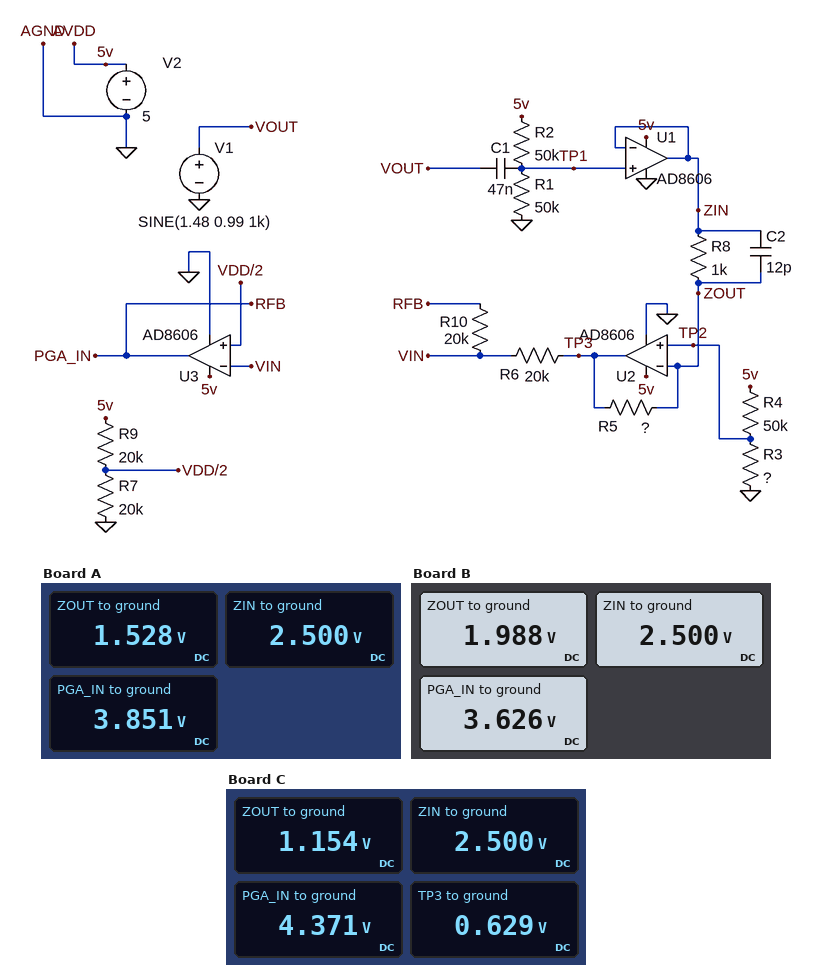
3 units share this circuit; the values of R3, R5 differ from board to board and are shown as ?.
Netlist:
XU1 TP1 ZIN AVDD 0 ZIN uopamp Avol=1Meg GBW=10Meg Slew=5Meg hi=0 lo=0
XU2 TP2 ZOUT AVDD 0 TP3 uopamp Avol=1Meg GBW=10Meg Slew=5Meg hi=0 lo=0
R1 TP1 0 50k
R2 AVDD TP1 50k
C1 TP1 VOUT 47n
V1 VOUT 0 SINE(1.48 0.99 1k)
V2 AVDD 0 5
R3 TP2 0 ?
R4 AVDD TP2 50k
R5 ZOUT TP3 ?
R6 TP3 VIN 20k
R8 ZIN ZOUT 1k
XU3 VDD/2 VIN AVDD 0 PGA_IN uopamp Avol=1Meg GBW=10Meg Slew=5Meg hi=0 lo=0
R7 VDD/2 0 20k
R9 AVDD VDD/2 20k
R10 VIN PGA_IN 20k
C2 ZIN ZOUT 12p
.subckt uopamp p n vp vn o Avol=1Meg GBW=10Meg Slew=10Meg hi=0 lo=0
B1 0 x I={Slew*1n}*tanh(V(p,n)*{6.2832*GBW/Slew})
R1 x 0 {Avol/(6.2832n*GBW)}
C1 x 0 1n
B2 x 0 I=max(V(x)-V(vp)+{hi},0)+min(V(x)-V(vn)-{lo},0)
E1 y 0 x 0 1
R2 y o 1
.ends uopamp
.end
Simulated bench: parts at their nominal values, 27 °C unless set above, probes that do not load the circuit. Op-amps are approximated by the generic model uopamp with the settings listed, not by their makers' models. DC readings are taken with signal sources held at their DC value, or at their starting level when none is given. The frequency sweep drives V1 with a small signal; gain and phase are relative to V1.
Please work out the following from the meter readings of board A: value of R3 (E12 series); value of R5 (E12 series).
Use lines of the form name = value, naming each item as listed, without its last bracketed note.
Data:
value of R3 = 22 kΩ
value of R5 = 390 Ω
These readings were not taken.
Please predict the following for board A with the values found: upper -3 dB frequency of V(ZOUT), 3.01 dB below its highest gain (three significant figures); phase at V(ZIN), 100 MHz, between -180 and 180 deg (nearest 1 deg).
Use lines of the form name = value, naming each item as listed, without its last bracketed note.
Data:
upper -3 dB frequency of V(ZOUT), 3.01 dB below its highest gain = 47.1 MHz
phase at V(ZIN), 100 MHz, between -180 and 180 deg = -84 deg
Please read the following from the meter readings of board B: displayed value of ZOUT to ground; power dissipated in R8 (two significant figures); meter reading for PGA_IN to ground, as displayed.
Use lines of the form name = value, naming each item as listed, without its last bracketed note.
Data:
displayed value of ZOUT to ground = 1.988 V
power dissipated in R8 = 260 µW
meter reading for PGA_IN to ground, as displayed = 3.626 V
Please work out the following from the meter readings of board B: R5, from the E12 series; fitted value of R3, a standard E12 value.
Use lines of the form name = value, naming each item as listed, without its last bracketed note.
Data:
R5, from the E12 series = 1.2 kΩ
fitted value of R3, a standard E12 value = 33 kΩ
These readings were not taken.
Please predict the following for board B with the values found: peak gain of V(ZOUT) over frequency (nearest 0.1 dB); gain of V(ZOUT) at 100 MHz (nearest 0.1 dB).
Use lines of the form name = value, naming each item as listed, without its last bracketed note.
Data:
peak gain of V(ZOUT) over frequency = -6.3 dB
gain of V(ZOUT) at 100 MHz = -20.1 dB
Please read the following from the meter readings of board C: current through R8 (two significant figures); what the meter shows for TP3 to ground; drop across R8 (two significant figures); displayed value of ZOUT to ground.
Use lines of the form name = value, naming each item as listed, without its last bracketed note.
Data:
current through R8 = 1.3 mA
what the meter shows for TP3 to ground = 0.629 V
drop across R8 = 1.3 V
displayed value of ZOUT to ground = 1.154 V
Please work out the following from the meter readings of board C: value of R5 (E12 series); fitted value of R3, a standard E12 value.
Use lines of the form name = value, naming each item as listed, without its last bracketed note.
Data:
value of R5 = 390 Ω
fitted value of R3, a standard E12 value = 15 kΩ
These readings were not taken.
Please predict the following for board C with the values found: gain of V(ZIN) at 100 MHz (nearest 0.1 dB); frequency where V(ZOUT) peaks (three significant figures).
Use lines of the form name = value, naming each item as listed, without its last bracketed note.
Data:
gain of V(ZIN) at 100 MHz = -20.1 dB
frequency where V(ZOUT) peaks = 14.8 MHz
